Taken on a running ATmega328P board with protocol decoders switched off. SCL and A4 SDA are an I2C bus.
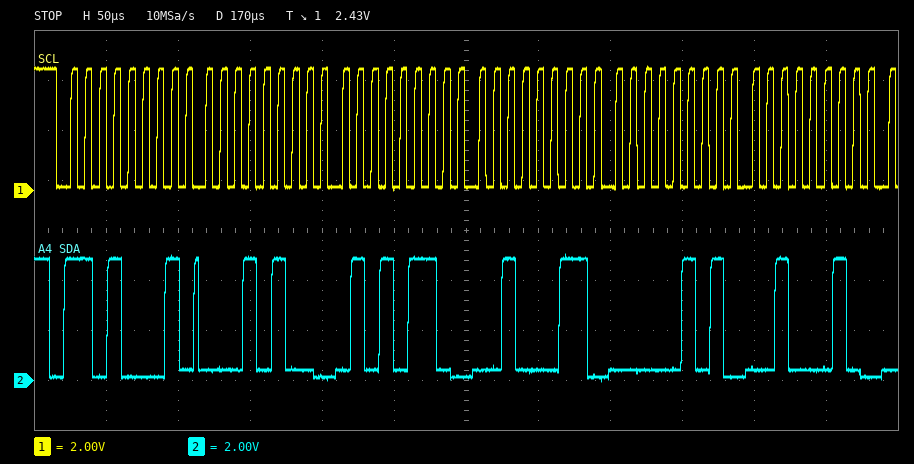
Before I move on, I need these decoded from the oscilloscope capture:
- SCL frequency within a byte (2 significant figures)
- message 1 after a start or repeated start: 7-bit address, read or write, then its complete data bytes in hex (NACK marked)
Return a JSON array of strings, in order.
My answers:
["100 kHz", "0x68 read: 14 56 23 05 22"]
